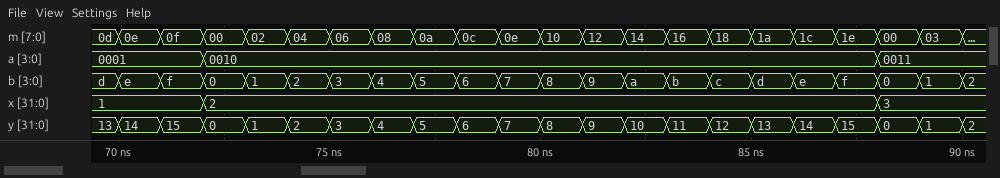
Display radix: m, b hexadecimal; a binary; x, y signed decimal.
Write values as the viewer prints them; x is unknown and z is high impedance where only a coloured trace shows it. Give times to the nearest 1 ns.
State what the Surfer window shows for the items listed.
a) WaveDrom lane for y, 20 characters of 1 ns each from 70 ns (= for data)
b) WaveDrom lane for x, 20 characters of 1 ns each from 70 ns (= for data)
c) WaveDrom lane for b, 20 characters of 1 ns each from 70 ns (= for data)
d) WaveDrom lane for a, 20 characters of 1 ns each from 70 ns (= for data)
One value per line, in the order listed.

{name: 'y', wave: '====================', data: '14 15 0 1 2 3 4 5 6 7 8 9 10 11 12 13 14 15 0 1'}
{name: 'x', wave: '=.=...............=.', data: '1 2 3'}
{name: 'b', wave: '====================', data: 'e f 0 1 2 3 4 5 6 7 8 9 a b c d e f 0 1'}
{name: 'a', wave: '=.=...............=.', data: '0001 0010 0011'}
